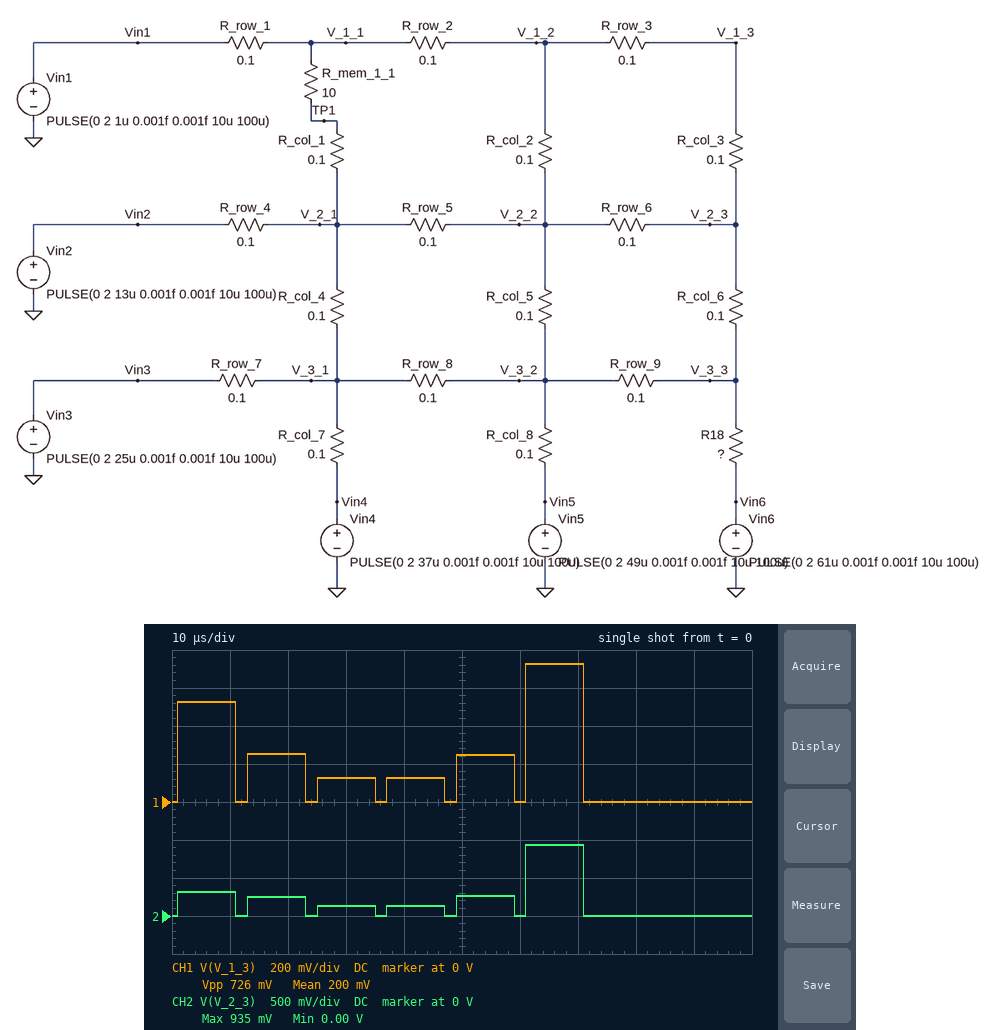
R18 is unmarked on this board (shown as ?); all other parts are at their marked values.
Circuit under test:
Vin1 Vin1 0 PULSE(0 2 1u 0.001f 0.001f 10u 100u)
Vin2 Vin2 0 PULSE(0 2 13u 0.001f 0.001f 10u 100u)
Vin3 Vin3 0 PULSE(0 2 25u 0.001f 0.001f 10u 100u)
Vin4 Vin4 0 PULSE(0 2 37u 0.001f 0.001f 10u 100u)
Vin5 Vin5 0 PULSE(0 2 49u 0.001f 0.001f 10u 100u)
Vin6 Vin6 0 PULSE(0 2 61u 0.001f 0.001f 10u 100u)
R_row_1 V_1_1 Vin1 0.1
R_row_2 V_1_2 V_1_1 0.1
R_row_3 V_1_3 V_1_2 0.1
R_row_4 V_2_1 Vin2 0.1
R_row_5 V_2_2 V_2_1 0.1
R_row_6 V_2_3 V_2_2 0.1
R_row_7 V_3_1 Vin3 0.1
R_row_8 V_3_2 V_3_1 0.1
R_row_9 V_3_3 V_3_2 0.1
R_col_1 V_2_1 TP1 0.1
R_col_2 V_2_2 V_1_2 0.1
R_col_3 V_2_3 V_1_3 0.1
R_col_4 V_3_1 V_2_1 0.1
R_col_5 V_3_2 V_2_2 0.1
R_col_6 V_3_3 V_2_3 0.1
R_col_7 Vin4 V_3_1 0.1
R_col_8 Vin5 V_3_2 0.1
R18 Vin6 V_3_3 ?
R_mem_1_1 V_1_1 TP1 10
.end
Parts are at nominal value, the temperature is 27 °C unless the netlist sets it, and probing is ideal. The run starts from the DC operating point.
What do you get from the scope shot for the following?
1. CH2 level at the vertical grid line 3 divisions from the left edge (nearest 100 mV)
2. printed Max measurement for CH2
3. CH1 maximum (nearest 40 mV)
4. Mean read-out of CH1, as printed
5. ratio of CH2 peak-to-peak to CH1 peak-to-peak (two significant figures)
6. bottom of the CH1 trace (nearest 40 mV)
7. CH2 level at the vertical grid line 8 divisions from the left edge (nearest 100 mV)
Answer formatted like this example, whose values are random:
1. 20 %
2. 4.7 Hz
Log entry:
1. 100 mV
2. 935 mV
3. 720 mV
4. 200 mV
5. 1.3
6. 0 V
7. 0 V
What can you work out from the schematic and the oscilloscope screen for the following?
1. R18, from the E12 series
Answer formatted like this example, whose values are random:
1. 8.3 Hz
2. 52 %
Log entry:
1. 0.033 Ω
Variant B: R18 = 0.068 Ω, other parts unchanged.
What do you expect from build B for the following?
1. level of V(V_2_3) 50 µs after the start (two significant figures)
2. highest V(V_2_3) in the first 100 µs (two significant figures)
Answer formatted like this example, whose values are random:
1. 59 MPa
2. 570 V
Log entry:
1. 330 mV
2. 740 mV
